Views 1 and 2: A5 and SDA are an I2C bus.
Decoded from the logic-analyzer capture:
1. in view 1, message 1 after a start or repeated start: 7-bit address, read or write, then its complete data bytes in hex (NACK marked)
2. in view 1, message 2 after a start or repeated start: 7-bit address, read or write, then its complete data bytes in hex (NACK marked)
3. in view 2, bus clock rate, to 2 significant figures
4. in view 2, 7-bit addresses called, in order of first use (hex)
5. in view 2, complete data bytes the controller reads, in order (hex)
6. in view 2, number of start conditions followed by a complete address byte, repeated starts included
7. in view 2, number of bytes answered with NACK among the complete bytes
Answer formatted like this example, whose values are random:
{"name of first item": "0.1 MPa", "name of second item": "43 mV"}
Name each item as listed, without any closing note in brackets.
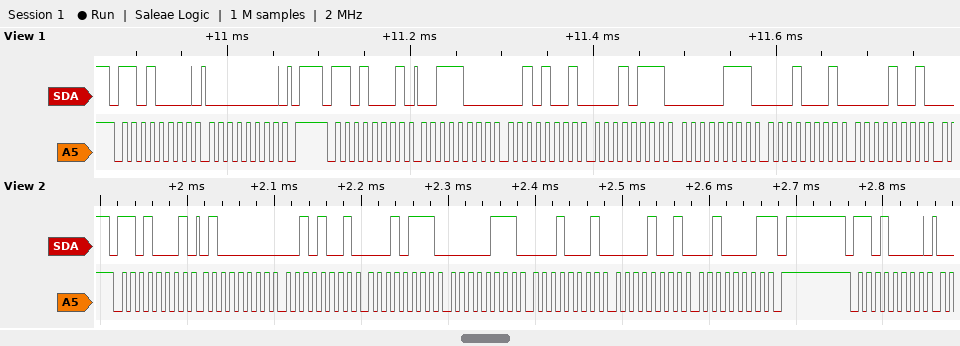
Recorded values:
{"in view 1, message 1 after a start or repeated start: 7-bit address, read or write, then its complete data bytes in hex": "0x68 write: 00", "in view 1, message 2 after a start or repeated start: 7-bit address, read or write, then its complete data bytes in hex": "0x68 read: 38 29 17 07 11 09", "in view 2, bus clock rate, to 2 significant figures": "100 kHz", "in view 2, 7-bit addresses called, in order of first use": "0x68", "in view 2, complete data bytes the controller reads, in order": "40 29 17 07 11 09 21", "in view 2, number of start conditions followed by a complete address byte, repeated starts included": "2", "in view 2, number of bytes answered with NACK among the complete bytes": "1"}
